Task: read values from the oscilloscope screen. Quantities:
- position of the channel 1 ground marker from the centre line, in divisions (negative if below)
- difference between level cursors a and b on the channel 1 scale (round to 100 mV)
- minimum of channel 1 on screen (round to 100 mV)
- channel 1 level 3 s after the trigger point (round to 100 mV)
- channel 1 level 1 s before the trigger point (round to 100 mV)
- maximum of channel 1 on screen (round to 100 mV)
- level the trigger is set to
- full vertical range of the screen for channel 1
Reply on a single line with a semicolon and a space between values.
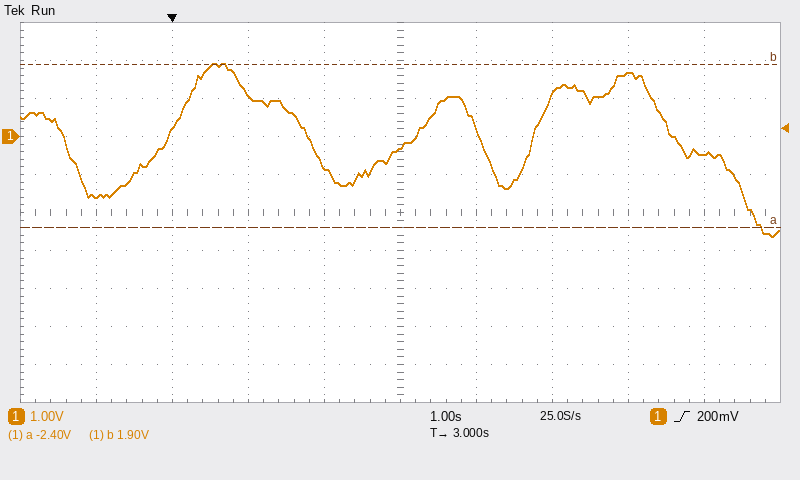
+2.0 div; 4.3 V; -2.6 V; -300 mV; -1.6 V; 1.9 V; 200 mV; 10 V
